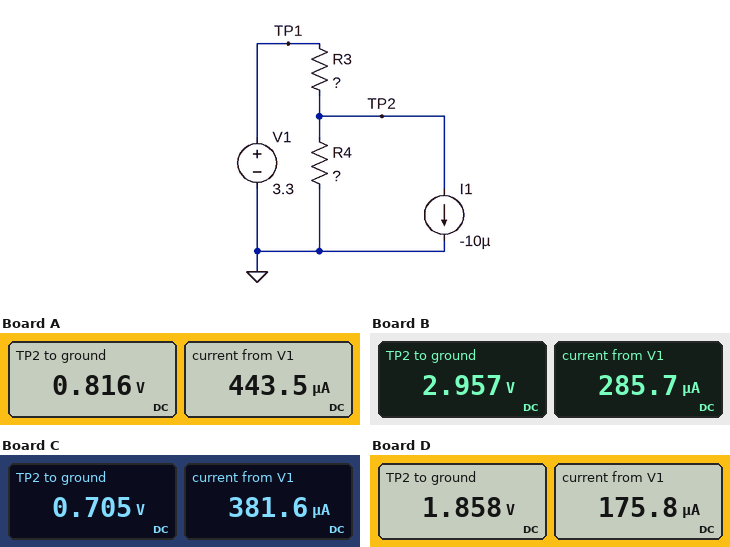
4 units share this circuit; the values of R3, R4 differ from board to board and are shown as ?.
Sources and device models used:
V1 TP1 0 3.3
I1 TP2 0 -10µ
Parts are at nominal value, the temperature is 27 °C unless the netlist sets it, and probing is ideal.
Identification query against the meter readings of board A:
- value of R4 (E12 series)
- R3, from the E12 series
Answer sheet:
1.8 kΩ
5.6 kΩ
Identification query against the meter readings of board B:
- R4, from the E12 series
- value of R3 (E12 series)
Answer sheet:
10 kΩ
1.2 kΩ
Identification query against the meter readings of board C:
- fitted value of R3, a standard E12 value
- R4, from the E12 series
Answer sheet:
6.8 kΩ
1.8 kΩ
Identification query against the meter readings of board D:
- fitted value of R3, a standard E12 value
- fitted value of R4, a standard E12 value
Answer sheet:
8.2 kΩ
10 kΩ
